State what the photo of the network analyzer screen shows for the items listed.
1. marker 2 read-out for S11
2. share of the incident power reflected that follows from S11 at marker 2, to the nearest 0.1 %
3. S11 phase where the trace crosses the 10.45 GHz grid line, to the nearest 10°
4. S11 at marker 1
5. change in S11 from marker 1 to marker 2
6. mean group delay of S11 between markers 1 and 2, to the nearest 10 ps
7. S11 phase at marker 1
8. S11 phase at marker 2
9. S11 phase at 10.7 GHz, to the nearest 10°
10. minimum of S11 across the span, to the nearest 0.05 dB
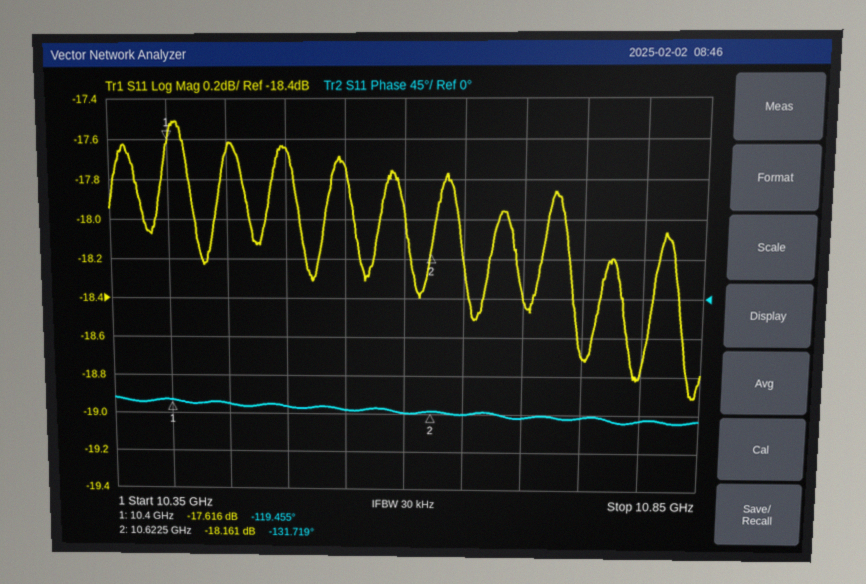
-18.161 dB
1.5 %
-120°
-17.616 dB
-0.545 dB
150 ps
-119.455°
-131.719°
-140°
-18.90 dB
